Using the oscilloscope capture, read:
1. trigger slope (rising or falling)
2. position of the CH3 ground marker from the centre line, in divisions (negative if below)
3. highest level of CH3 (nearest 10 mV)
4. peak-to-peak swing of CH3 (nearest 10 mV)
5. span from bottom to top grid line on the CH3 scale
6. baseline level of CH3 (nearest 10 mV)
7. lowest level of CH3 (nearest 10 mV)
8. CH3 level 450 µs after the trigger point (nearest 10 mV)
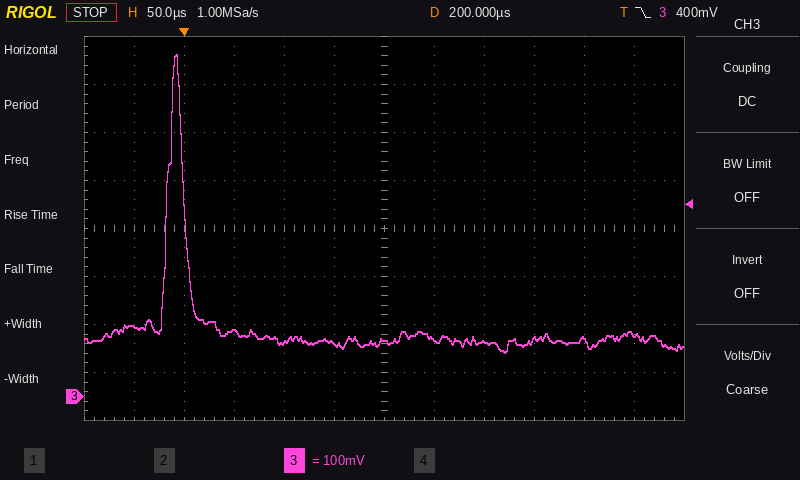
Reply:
falling
-3.5 div
710 mV
620 mV
800 mV
120 mV
90 mV
130 mV
